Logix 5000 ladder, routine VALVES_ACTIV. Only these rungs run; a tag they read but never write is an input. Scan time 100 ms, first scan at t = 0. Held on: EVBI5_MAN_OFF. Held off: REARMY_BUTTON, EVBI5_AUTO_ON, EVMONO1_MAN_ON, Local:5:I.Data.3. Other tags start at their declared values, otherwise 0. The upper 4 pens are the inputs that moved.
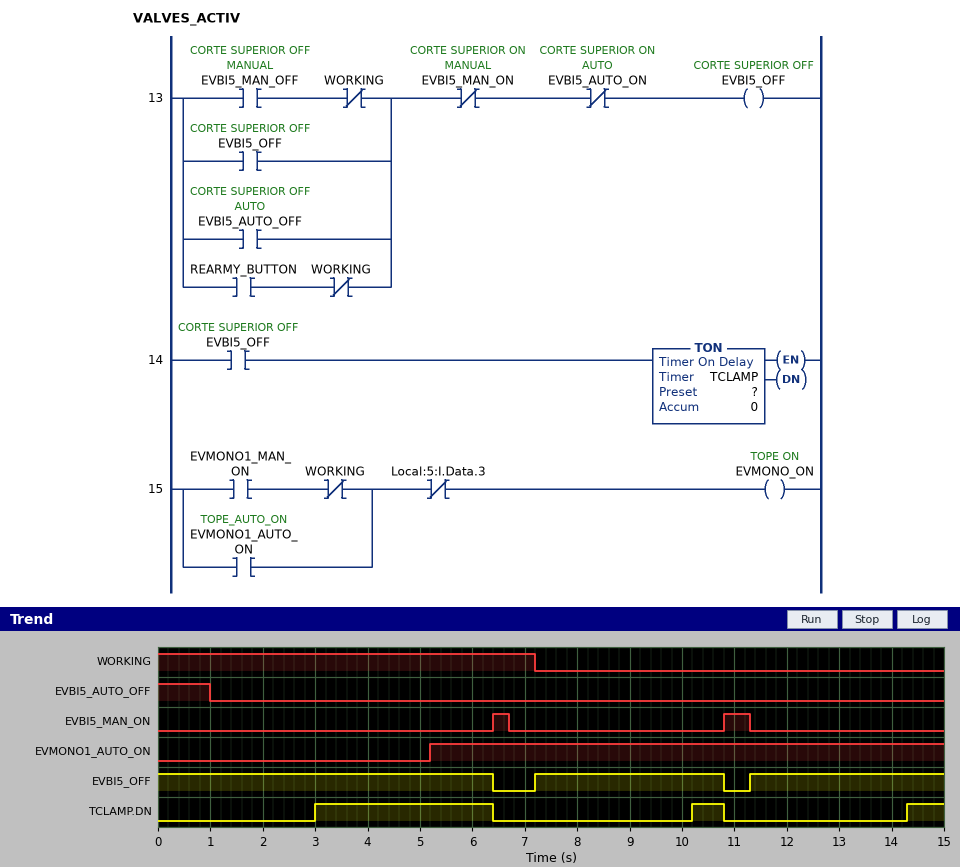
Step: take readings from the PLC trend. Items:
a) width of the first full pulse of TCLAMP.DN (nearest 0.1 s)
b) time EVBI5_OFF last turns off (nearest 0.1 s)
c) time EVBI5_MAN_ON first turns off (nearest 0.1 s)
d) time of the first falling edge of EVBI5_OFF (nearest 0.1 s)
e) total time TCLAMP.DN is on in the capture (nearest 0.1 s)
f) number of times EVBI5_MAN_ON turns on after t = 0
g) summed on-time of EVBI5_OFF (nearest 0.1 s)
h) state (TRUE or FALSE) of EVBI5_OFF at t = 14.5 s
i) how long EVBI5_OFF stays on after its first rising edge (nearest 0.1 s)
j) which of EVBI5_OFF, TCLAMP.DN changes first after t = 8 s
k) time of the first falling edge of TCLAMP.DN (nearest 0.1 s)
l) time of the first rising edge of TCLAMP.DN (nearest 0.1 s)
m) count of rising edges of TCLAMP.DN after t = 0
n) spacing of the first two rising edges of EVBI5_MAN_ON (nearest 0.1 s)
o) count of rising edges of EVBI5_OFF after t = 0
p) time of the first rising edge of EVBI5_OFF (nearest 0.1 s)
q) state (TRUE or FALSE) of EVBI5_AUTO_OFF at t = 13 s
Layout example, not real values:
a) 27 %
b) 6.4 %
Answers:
a) 3.4 s
b) 10.8 s
c) 6.7 s
d) 6.4 s
e) 4.7 s
f) 2
g) 13.7 s
h) TRUE
i) 3.6 s
j) TCLAMP.DN
k) 6.4 s
l) 3.0 s
m) 3
n) 4.4 s
o) 2
p) 7.2 s
q) FALSE
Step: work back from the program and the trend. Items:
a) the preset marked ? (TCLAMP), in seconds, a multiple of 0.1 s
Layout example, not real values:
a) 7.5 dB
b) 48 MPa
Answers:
a) 3.0 s
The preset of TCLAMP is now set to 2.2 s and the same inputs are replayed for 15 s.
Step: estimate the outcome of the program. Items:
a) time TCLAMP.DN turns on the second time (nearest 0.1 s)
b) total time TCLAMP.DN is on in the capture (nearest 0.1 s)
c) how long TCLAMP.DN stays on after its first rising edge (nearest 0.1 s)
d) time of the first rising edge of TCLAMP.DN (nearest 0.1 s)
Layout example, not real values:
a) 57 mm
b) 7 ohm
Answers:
a) 9.4 s
b) 7.1 s
c) 4.2 s
d) 2.2 s
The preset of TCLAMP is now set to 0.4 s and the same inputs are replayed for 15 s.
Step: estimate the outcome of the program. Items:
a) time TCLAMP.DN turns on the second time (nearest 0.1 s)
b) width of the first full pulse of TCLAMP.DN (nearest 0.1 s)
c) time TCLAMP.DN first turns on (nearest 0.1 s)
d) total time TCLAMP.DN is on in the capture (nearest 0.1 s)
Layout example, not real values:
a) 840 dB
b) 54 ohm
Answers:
a) 7.6 s
b) 6.0 s
c) 0.4 s
d) 12.5 s
